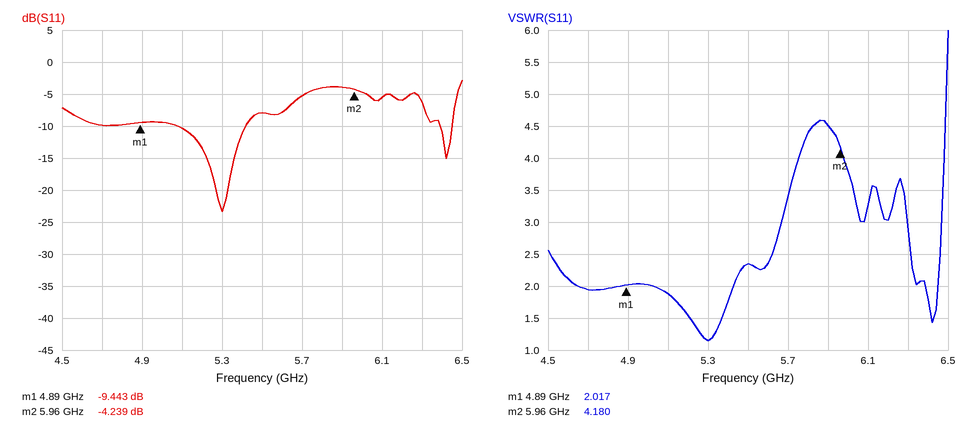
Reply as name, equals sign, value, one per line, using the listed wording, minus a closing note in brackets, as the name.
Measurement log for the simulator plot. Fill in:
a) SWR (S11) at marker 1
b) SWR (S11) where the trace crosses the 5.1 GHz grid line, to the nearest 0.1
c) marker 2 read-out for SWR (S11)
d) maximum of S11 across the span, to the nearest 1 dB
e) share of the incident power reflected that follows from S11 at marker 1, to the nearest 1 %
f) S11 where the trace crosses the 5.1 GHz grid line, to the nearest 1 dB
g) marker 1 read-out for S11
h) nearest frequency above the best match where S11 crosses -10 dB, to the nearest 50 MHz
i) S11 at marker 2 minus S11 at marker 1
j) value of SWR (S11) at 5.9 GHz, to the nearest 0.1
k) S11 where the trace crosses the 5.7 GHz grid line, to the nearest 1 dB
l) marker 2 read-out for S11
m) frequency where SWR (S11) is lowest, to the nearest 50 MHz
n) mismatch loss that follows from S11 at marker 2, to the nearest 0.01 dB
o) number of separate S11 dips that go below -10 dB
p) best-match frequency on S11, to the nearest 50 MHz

SWR (S11) at marker 1 = 2.017
SWR (S11) where the trace crosses the 5.1 GHz grid line, to the nearest 0.1 = 1.9
marker 2 read-out for SWR = 4.180
maximum of S11 across the span, to the nearest 1 dB = -3 dB
share of the incident power reflected that follows from S11 at marker 1, to the nearest 1 % = 11 %
S11 where the trace crosses the 5.1 GHz grid line, to the nearest 1 dB = -10 dB
marker 1 read-out for S11 = -9.443 dB
nearest frequency above the best match where S11 crosses -10 dB, to the nearest 50 MHz = 5.40 GHz
S11 at marker 2 minus S11 at marker 1 = 5.204 dB
value of SWR (S11) at 5.9 GHz, to the nearest 0.1 = 4.5
S11 where the trace crosses the 5.7 GHz grid line, to the nearest 1 dB = -5 dB
marker 2 read-out for S11 = -4.239 dB
frequency where SWR (S11) is lowest, to the nearest 50 MHz = 5.30 GHz
mismatch loss that follows from S11 at marker 2, to the nearest 0.01 dB = 2.05 dB
number of separate S11 dips that go below -10 dB = 2
best-match frequency on S11, to the nearest 50 MHz = 5.30 GHz
